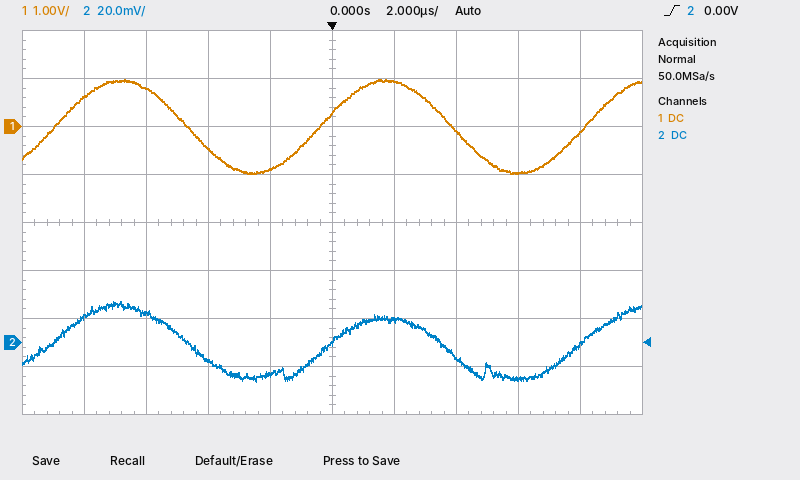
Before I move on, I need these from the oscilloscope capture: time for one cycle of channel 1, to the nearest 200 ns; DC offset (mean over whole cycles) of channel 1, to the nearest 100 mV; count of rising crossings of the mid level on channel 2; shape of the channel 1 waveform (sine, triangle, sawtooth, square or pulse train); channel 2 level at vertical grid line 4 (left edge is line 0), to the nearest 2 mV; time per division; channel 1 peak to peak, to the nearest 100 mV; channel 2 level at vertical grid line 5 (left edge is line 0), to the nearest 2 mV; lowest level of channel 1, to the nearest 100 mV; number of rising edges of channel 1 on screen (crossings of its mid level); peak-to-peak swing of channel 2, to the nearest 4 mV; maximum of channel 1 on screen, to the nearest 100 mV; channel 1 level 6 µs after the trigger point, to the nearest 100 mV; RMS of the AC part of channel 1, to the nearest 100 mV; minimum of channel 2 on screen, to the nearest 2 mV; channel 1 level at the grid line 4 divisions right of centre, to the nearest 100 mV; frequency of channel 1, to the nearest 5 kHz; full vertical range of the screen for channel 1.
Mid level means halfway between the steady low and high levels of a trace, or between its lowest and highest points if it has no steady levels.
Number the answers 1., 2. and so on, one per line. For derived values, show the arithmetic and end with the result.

1. 8.6 µs
2. (1.0 V + (-1.0 V)) / 2 ≈ 0.0 V
3. 3
4. sine
5. -14 mV
6. 2 µs
7. 1.0 V − (-1.0 V) = 2.0 V
8. 0 mV
9. -1.0 V
10. 3
11. 32 mV
12. 1.0 V
13. -1.0 V
14. 2.0 V / (2√2) ≈ 707 mV, so 700 mV to the nearest 100 mV
15. -16 mV
16. -100 mV
17. 1 / 8.6 µs ≈ 116 kHz, so 115 kHz to the nearest 5 kHz
18. 8 V
